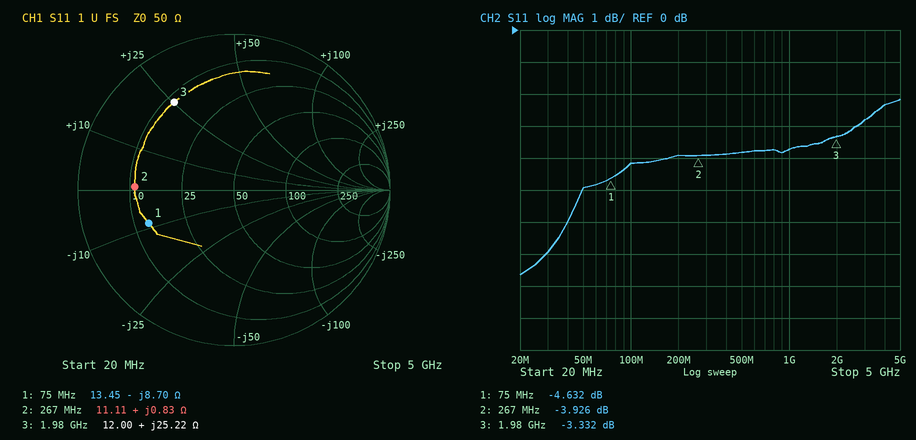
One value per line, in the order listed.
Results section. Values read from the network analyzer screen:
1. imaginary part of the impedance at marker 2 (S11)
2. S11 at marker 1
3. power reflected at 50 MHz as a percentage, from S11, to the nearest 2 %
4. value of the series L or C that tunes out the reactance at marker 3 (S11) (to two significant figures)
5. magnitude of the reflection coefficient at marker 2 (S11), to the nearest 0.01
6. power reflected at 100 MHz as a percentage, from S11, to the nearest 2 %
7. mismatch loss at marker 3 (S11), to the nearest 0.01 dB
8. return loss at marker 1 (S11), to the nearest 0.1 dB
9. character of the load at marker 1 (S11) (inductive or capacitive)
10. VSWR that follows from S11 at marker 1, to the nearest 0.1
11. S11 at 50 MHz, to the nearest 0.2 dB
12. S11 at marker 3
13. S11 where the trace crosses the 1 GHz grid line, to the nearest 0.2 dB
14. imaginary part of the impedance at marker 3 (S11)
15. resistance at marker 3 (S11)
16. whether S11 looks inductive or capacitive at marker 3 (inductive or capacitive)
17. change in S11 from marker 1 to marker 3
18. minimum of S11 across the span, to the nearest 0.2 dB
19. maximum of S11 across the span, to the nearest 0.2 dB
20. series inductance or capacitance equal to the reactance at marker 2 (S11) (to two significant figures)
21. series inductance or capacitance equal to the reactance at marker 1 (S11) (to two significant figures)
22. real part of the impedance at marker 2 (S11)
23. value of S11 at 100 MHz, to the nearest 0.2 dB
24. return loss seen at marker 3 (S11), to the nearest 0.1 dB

+0.83 Ω
-4.632 dB
32 %
3.2 pF
0.64
38 %
2.71 dB
4.6 dB
capacitive
3.8
-5.0 dB
-3.332 dB
-3.8 dB
+25.22 Ω
12.00 Ω
inductive
1.300 dB
-7.6 dB
-2.2 dB
490 pH
240 pF
11.11 Ω
-4.2 dB
3.3 dB
